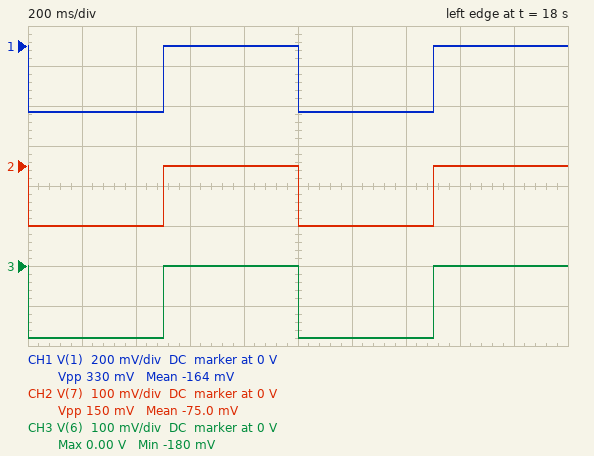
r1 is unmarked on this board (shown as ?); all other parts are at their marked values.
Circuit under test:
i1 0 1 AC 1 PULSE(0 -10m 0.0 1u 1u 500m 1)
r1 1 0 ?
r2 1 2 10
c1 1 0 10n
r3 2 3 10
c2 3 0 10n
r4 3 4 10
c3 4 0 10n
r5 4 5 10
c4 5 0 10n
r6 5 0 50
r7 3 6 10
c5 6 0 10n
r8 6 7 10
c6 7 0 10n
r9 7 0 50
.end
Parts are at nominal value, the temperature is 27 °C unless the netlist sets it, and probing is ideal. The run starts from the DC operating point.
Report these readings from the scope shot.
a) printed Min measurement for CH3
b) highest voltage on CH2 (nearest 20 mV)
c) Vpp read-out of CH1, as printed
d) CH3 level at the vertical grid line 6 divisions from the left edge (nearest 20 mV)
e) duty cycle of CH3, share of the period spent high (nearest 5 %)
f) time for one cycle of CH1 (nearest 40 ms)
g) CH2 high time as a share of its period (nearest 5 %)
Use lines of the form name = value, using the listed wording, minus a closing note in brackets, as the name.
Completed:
printed Min measurement for CH3 = -180 mV
highest voltage on CH2 = 0 V
Vpp read-out of CH1, as printed = 330 mV
CH3 level at the vertical grid line 6 divisions from the left edge = -180 mV
duty cycle of CH3, share of the period spent high = 50 %
time for one cycle of CH1 = 1.00 s
CH2 high time as a share of its period = 50 %
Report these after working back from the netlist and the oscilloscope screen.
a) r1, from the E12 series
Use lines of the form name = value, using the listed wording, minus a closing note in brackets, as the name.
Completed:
r1, from the E12 series = 82 Ω
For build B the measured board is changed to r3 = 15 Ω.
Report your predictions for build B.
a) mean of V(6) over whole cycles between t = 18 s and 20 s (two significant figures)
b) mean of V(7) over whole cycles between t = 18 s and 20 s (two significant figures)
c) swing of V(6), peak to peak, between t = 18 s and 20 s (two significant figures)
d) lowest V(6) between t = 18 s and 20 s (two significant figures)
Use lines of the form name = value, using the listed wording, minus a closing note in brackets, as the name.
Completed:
mean of V(6) over whole cycles between t = 18 s and 20 s = -87 mV
mean of V(7) over whole cycles between t = 18 s and 20 s = -72 mV
swing of V(6), peak to peak, between t = 18 s and 20 s = 170 mV
lowest V(6) between t = 18 s and 20 s = -170 mV
